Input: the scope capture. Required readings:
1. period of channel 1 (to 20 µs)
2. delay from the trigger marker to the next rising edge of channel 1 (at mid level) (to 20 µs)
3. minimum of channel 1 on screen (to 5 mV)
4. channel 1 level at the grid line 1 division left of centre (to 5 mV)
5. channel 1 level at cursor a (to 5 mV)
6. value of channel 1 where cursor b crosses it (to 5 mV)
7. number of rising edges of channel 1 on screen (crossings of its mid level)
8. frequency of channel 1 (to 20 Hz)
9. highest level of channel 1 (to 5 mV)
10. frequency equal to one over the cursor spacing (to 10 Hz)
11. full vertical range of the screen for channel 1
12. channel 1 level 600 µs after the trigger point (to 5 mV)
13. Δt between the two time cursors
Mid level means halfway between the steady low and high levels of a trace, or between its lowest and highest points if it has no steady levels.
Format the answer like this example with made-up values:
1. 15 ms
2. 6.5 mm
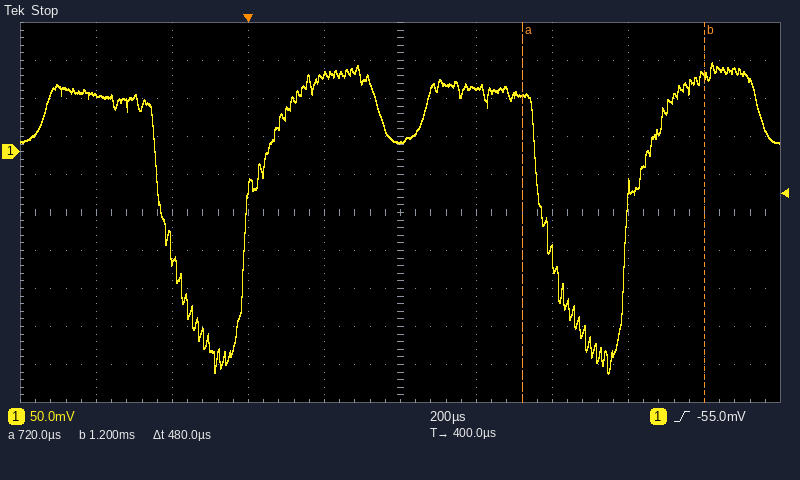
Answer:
1. 1.00 ms
2. 1.00 ms
3. -290 mV
4. 100 mV
5. 75 mV
6. 100 mV
7. 2
8. 1.00 kHz
9. 115 mV
10. 2.08 kHz
11. 500 mV
12. 85 mV
13. 480 µs
